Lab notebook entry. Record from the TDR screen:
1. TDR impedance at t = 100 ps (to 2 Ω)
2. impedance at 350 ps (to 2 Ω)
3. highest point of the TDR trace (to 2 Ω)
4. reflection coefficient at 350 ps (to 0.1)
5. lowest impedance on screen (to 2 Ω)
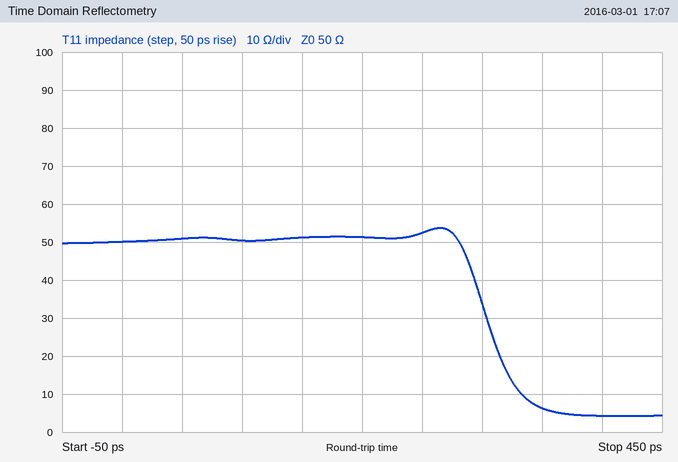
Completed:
50 Ω
6 Ω
54 Ω
-0.8
4 Ω
